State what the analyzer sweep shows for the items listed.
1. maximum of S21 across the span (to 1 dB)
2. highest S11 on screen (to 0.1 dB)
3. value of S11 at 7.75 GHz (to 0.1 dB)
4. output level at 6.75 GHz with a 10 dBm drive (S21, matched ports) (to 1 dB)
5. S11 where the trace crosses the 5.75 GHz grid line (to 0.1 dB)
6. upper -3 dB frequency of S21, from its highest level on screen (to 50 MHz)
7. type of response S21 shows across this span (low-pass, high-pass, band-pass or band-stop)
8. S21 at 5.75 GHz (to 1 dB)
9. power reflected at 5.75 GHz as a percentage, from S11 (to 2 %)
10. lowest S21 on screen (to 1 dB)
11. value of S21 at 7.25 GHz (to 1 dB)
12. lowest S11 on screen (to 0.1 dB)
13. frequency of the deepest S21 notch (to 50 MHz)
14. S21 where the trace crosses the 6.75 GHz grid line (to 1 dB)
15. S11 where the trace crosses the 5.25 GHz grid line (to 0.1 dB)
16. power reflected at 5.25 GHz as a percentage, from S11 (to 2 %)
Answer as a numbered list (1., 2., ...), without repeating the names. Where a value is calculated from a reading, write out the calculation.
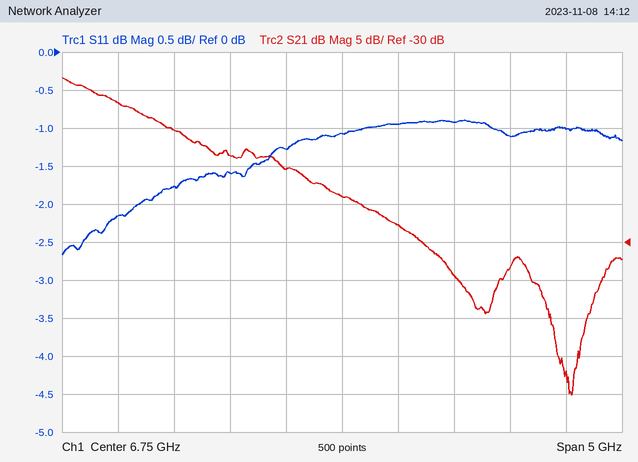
1. -8 dB
2. -0.9 dB
3. -0.9 dB
4. 10 dBm + (-24 dB) = -14 dBm
5. -1.6 dB
6. 4.70 GHz
7. low-pass
8. -19 dB
9. 10^(-1.6/10) ≈ 69.2 %, so 70 % to the nearest 2 %
10. -50 dB
11. -28 dB
12. -2.7 dB
13. 8.80 GHz
14. -24 dB
15. -1.8 dB
16. 10^(-1.8/10) ≈ 66 %
